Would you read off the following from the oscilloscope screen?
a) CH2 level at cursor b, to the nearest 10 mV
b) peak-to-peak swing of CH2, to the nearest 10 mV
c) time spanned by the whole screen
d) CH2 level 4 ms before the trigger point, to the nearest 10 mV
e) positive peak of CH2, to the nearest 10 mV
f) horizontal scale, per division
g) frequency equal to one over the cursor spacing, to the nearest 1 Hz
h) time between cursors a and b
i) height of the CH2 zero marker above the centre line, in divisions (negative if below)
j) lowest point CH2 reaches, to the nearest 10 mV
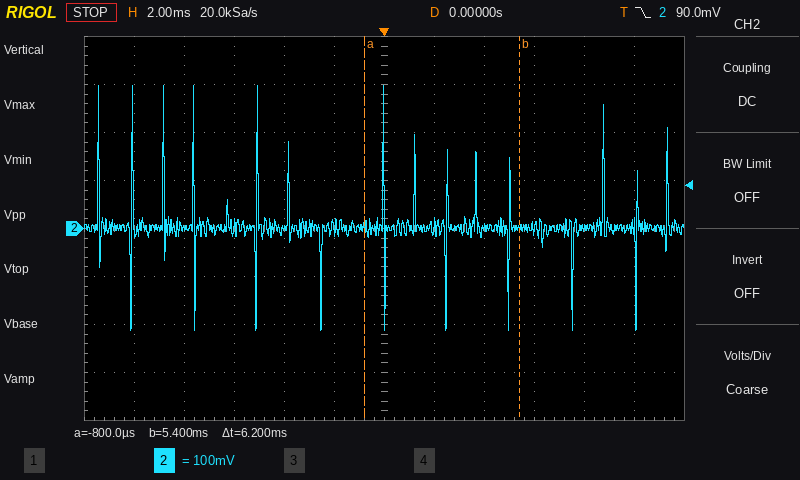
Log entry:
0 mV
510 mV
24 ms
0 mV
300 mV
2 ms
161 Hz
6.2 ms
0.0 div
-210 mV
